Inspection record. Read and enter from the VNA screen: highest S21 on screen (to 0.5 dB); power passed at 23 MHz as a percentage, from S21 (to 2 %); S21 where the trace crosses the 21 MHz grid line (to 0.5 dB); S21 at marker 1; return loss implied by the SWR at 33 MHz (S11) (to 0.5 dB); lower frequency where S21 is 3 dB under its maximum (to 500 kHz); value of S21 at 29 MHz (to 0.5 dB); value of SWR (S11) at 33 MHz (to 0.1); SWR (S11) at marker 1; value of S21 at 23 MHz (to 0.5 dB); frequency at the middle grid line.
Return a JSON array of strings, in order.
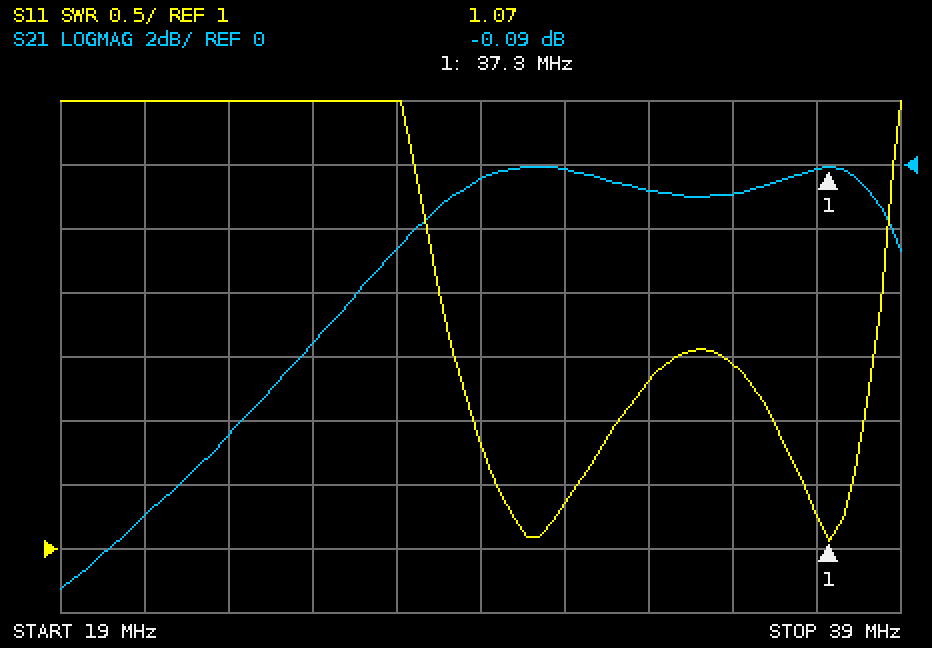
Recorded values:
["0.0 dB", "14 %", "-11.0 dB", "-0.09 dB", "8.0 dB", "26.5 MHz", "-0.5 dB", "2.3", "1.07", "-8.5 dB", "29 MHz"]
